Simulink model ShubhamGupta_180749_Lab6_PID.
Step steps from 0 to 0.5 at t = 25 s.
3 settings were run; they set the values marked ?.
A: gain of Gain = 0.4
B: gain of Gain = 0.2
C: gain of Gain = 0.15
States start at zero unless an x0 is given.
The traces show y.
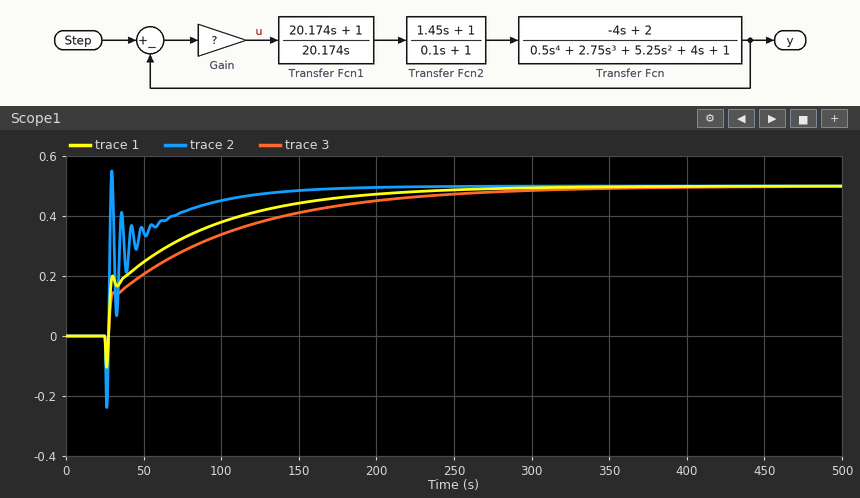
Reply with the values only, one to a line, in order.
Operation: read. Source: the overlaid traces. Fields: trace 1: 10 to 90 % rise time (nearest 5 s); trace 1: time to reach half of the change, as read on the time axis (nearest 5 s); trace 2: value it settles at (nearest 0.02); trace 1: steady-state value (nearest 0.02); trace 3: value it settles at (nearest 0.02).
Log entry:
130 s
50 s
0.50
0.50
0.50
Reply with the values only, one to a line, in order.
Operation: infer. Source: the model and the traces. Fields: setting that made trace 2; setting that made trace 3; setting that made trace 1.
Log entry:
A
C
B
